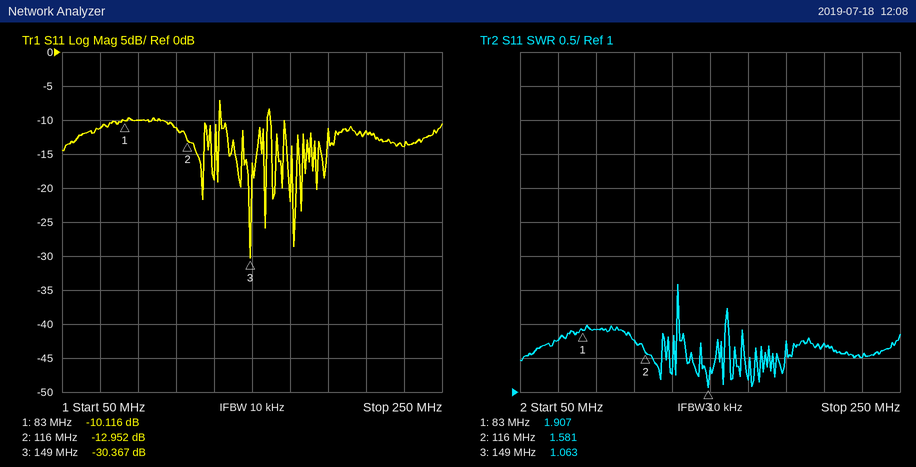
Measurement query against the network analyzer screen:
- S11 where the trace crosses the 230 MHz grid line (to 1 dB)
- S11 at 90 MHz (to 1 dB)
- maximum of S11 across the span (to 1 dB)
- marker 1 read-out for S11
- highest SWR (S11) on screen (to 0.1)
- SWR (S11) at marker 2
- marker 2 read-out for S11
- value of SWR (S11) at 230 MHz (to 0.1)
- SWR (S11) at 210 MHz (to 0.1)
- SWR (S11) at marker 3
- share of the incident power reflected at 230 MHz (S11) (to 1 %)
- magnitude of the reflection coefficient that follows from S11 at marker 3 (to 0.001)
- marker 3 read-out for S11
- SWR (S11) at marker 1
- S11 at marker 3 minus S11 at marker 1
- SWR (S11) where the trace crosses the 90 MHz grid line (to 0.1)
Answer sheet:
-14 dB
-10 dB
-7 dB
-10.116 dB
2.6
1.581
-12.952 dB
1.5
1.7
1.063
4 %
0.030
-30.367 dB
1.907
-20.251 dB
1.9
